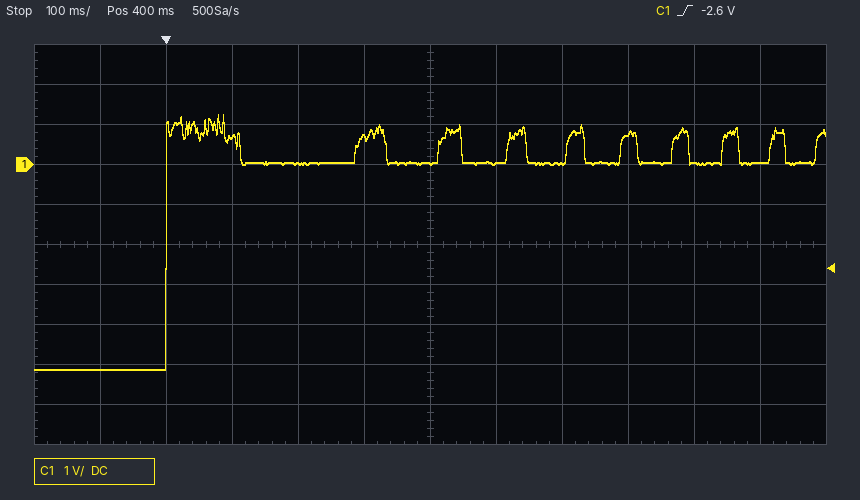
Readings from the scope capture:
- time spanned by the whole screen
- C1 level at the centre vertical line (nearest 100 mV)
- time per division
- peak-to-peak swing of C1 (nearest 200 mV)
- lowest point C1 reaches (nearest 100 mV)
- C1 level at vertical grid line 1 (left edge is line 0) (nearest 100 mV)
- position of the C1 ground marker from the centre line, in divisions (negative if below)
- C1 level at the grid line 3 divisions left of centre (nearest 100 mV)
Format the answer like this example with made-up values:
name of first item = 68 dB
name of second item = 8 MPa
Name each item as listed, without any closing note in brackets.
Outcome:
time spanned by the whole screen = 1.2 s
C1 level at the centre vertical line = 0.0 V
time per division = 100 ms
peak-to-peak swing of C1 = 6.4 V
lowest point C1 reaches = -5.1 V
C1 level at vertical grid line 1 (left edge is line 0) = -5.1 V
position of the C1 ground marker from the centre line, in divisions = +2.0 div
C1 level at the grid line 3 divisions left of centre = 700 mV
